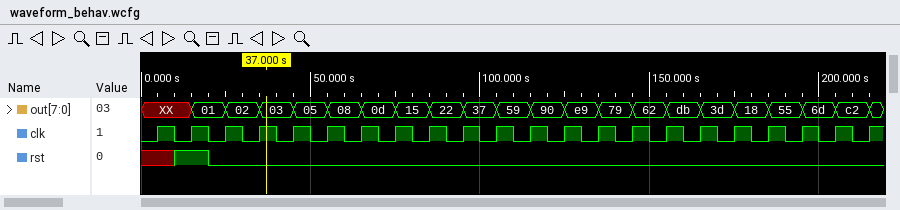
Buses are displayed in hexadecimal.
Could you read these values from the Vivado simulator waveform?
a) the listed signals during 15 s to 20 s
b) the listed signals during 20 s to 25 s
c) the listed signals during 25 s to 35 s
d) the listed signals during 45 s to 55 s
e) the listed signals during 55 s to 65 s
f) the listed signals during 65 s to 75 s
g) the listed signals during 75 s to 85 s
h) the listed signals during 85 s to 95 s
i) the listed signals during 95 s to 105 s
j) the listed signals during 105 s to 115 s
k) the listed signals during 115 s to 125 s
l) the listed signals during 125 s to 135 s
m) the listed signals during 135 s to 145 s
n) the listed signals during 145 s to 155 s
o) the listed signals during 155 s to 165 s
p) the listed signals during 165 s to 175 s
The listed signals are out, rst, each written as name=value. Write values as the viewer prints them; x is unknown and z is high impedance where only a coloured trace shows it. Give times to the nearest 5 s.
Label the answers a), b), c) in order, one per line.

a) out=01, rst=1
b) out=01, rst=0
c) out=02, rst=0
d) out=05, rst=0
e) out=08, rst=0
f) out=0d, rst=0
g) out=15, rst=0
h) out=22, rst=0
i) out=37, rst=0
j) out=59, rst=0
k) out=90, rst=0
l) out=e9, rst=0
m) out=79, rst=0
n) out=62, rst=0
o) out=db, rst=0
p) out=3d, rst=0
